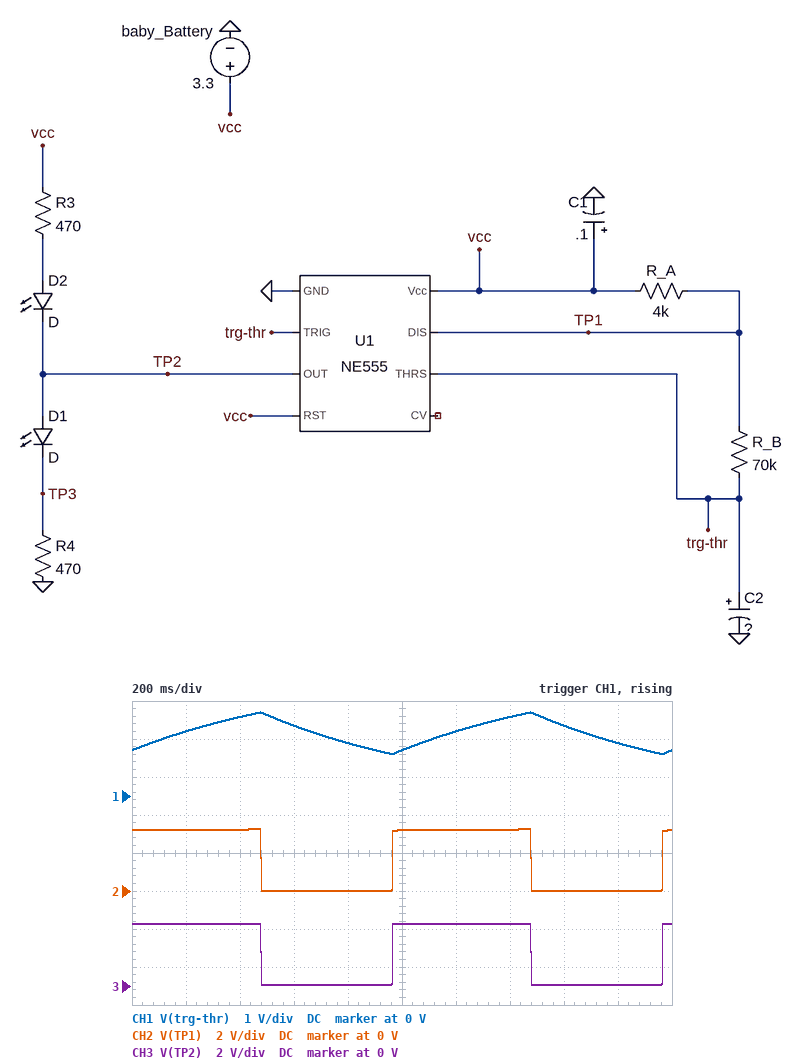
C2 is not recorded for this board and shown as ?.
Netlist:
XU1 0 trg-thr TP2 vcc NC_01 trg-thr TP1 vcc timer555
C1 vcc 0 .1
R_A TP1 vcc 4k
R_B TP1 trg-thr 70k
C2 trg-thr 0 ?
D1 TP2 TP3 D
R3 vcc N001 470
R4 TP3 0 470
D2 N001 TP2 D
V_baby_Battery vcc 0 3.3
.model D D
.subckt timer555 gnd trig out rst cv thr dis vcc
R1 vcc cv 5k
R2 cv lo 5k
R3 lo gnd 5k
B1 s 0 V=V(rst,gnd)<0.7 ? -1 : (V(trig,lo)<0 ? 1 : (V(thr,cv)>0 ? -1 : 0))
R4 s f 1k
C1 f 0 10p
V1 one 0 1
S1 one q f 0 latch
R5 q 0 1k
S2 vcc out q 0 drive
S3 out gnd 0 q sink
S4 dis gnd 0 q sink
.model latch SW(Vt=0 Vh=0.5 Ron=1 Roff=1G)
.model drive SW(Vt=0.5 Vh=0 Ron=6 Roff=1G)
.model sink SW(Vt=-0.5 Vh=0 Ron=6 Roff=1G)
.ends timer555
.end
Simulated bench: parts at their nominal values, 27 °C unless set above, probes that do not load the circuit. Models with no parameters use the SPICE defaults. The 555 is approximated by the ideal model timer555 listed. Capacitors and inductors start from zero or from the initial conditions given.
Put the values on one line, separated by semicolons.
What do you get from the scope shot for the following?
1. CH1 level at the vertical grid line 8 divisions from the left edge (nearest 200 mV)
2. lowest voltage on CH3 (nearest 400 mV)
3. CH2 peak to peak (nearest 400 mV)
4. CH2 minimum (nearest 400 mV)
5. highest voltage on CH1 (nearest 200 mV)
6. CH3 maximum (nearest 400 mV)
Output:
1.8 V; 0 V; 3.2 V; 0 V; 2.2 V; 3.2 V
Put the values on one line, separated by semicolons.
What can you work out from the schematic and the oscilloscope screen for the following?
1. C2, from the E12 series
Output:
10 µF
